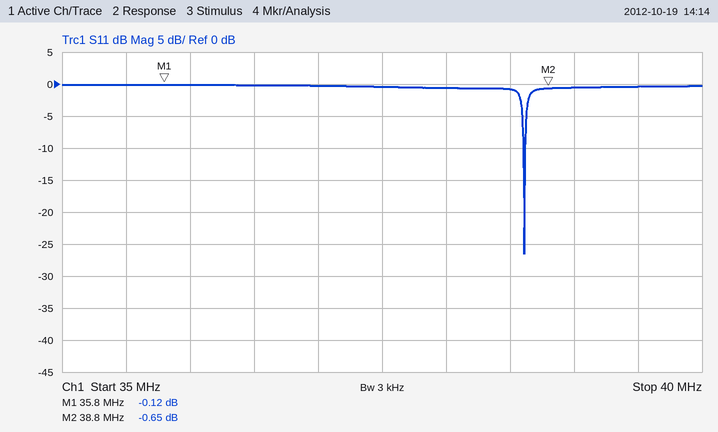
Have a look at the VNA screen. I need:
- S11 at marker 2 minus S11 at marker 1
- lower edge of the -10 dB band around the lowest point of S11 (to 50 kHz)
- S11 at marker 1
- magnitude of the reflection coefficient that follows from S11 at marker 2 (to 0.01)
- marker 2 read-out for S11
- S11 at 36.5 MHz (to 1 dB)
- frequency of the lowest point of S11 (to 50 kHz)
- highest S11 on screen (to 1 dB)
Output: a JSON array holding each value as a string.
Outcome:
["-0.53 dB", "38.60 MHz", "-0.12 dB", "0.93", "-0.65 dB", "0 dB", "38.60 MHz", "0 dB"]
